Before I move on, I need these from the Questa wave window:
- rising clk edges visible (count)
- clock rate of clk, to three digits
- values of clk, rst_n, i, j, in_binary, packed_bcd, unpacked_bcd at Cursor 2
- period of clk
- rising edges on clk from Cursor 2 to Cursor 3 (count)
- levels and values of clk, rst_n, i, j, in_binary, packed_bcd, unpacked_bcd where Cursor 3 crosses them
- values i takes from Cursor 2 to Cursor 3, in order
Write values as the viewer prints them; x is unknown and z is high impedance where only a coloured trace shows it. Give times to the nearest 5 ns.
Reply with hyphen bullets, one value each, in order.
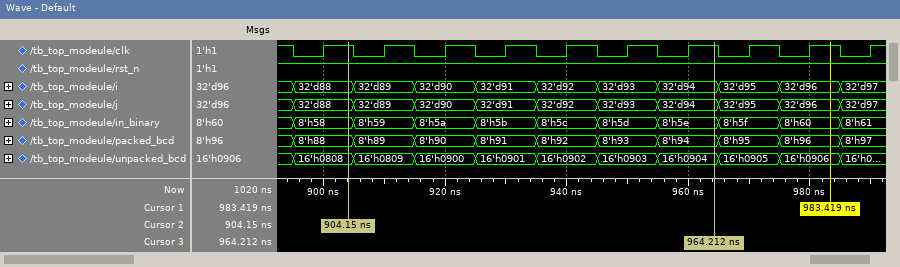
- 10
- 100 MHz
- clk=1, rst_n=1, i=32'd88, j=32'd88, in_binary=8'h58, packed_bcd=8'h88, unpacked_bcd=16'h0808
- 10 ns
- 6
- clk=1, rst_n=1, i=32'd94, j=32'd94, in_binary=8'h5e, packed_bcd=8'h94, unpacked_bcd=16'h0904
- 32'd88, 32'd89, 32'd90, 32'd91, 32'd92, 32'd93, 32'd94
